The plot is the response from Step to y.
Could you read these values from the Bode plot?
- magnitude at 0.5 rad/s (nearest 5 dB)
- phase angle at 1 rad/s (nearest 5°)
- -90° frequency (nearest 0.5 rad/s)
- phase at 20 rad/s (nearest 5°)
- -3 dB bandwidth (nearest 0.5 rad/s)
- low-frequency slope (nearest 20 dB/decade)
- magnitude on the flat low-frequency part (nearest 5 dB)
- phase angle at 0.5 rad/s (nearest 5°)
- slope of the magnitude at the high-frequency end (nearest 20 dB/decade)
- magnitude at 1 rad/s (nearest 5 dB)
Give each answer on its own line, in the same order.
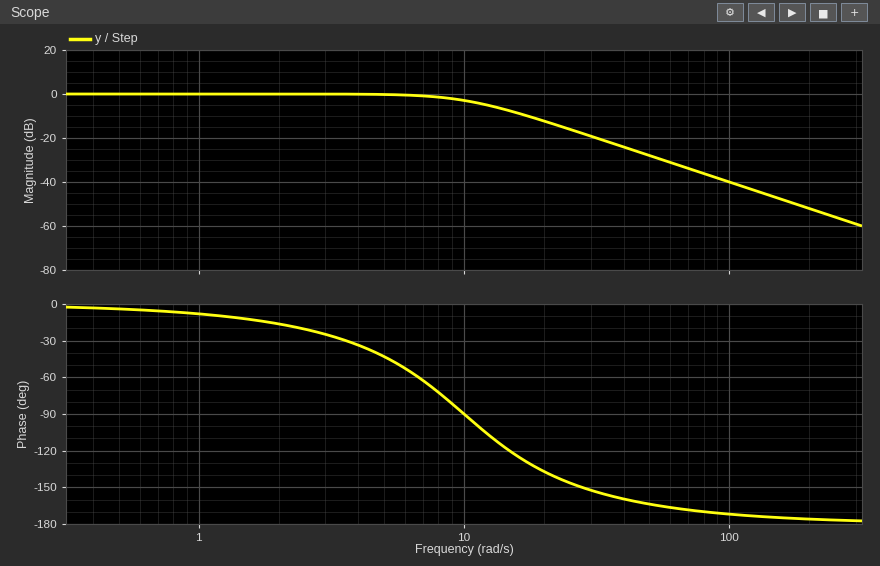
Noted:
0 dB
-10°
10.0 rad/s
-135°
10.0 rad/s
0 dB/decade
0 dB
-5°
-40 dB/decade
0 dB
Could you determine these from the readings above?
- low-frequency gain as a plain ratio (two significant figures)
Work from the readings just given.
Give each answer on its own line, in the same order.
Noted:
1.0
